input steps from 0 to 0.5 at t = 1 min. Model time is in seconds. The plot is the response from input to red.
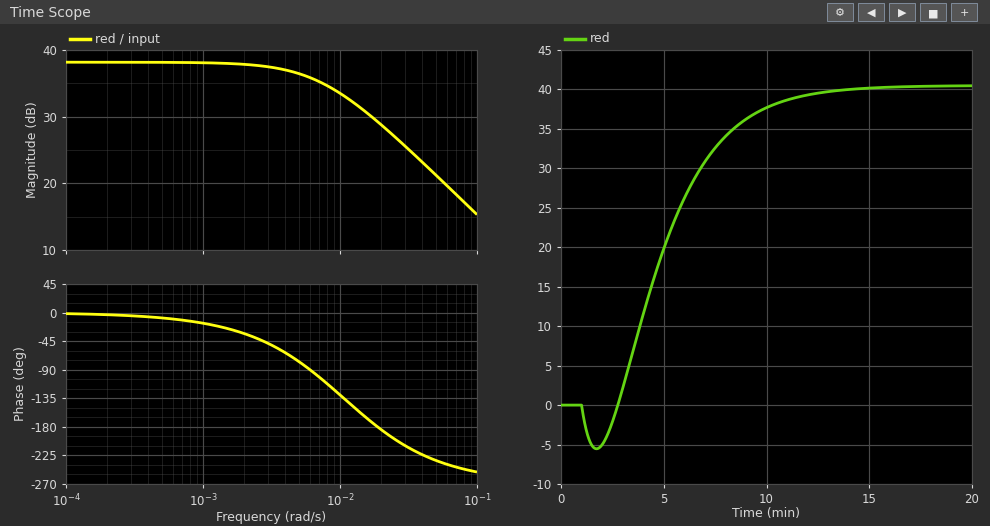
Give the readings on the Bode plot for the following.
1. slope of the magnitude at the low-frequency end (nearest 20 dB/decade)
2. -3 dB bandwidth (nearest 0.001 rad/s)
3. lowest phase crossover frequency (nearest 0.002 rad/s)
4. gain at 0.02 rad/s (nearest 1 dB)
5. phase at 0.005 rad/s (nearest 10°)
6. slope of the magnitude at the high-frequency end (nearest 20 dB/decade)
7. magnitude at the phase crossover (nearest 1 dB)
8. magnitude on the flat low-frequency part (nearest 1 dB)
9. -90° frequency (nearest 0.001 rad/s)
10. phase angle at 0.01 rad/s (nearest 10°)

0 dB/decade
0.007 rad/s
0.018 rad/s
29 dB
-80°
-20 dB/decade
29 dB
38 dB
0.006 rad/s
-130°
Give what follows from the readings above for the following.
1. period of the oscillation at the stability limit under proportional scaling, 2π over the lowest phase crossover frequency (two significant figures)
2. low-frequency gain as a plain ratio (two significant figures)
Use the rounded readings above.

350 s
79
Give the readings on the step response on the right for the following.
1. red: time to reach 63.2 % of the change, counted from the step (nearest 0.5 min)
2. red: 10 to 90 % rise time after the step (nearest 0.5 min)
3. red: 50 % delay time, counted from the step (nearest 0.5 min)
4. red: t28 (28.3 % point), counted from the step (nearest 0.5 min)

5.0 min
6.0 min
4.0 min
3.0 min
